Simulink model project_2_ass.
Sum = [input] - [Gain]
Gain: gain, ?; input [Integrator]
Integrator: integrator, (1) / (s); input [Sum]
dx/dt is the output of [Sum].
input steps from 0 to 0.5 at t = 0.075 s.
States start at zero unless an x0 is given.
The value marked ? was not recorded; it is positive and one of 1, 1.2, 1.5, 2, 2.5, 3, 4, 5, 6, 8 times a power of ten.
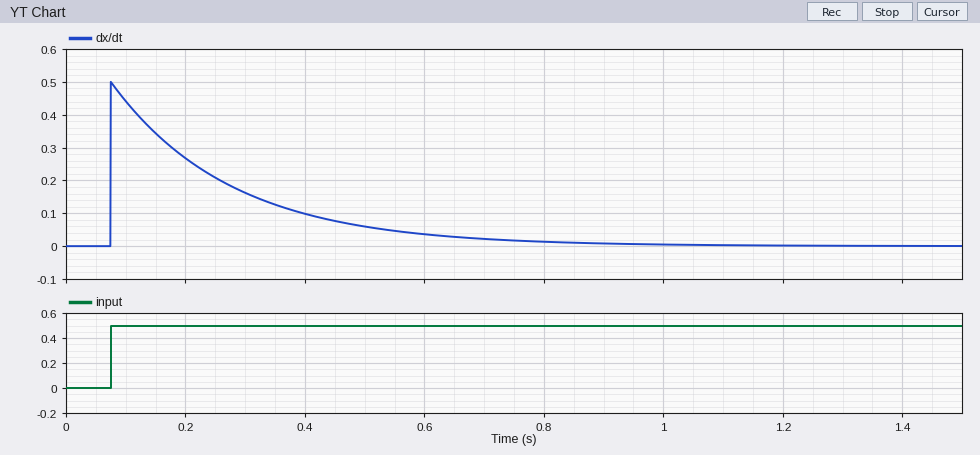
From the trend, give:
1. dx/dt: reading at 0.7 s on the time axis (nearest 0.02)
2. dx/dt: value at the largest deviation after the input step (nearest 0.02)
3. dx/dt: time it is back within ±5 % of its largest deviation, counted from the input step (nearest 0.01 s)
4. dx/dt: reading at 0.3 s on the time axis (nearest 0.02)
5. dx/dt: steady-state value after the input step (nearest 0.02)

0.02
0.50
0.60 s
0.16
0.00
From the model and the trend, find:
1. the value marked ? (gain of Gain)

5
